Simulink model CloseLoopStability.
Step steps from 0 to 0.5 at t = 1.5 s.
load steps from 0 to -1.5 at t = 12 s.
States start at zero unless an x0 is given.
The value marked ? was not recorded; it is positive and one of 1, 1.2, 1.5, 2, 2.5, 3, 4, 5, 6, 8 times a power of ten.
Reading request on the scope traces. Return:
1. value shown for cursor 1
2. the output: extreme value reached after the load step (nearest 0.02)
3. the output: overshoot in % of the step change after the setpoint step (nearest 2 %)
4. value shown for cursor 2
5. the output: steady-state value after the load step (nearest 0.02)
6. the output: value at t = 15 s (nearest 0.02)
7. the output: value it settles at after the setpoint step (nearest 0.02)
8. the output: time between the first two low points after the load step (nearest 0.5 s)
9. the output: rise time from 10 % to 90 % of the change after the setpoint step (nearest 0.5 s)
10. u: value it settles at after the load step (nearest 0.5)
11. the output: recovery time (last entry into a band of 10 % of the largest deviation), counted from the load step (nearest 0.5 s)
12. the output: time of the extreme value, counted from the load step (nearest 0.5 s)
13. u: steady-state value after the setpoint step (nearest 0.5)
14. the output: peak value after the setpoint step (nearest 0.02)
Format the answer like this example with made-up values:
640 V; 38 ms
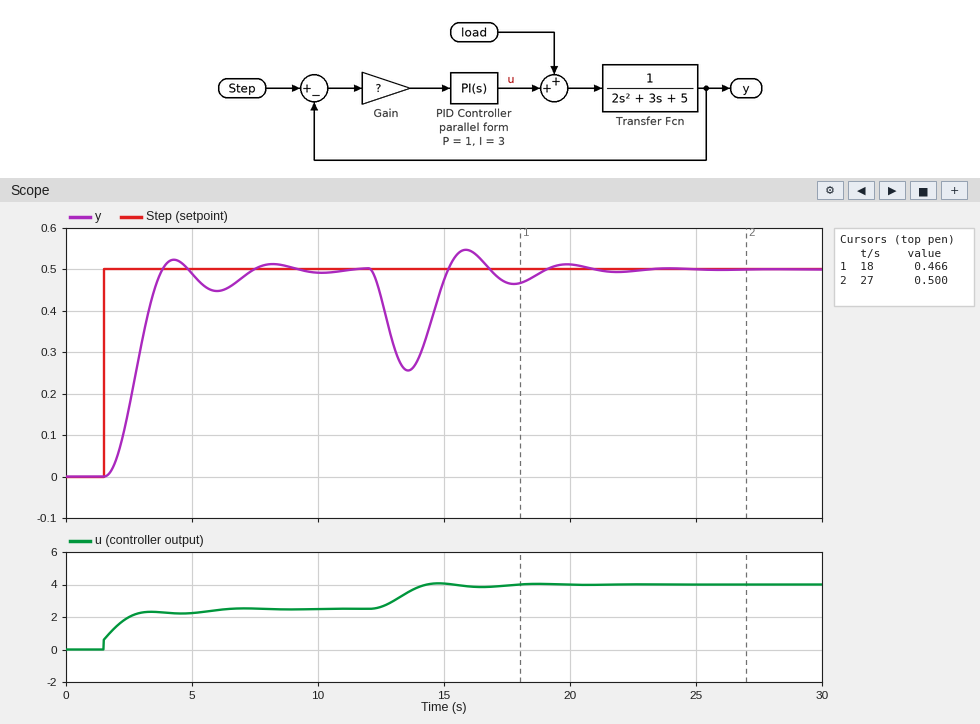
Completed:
0.466; 0.26; 4 %; 0.500; 0.50; 0.48; 0.50; 4.0 s; 1.5 s; 4.0; 6.5 s; 1.5 s; 2.5; 0.52
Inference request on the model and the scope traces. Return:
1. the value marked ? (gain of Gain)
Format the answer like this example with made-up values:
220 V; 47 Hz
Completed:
1.2
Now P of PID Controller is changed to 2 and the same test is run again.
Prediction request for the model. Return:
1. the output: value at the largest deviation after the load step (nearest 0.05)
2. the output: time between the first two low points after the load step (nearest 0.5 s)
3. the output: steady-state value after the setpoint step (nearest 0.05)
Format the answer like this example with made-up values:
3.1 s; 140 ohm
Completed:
0.30; 3.5 s; 0.50
